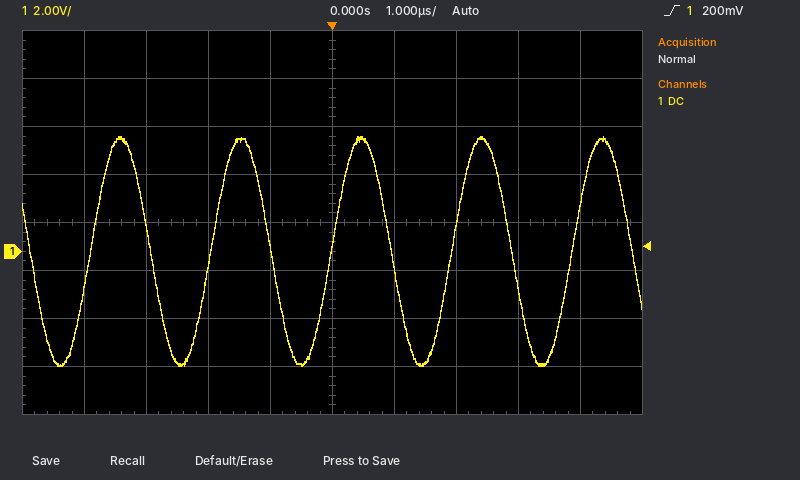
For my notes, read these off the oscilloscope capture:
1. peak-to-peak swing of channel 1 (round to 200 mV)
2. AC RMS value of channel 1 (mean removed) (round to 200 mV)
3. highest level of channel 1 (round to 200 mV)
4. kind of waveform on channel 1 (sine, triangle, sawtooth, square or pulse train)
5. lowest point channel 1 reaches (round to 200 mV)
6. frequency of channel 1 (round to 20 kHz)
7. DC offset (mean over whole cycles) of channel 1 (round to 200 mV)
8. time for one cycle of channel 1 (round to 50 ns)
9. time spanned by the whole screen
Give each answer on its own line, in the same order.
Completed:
9.6 V
3.4 V
4.8 V
sine
-4.8 V
520 kHz
0.0 V
1.95 µs
10 µs
